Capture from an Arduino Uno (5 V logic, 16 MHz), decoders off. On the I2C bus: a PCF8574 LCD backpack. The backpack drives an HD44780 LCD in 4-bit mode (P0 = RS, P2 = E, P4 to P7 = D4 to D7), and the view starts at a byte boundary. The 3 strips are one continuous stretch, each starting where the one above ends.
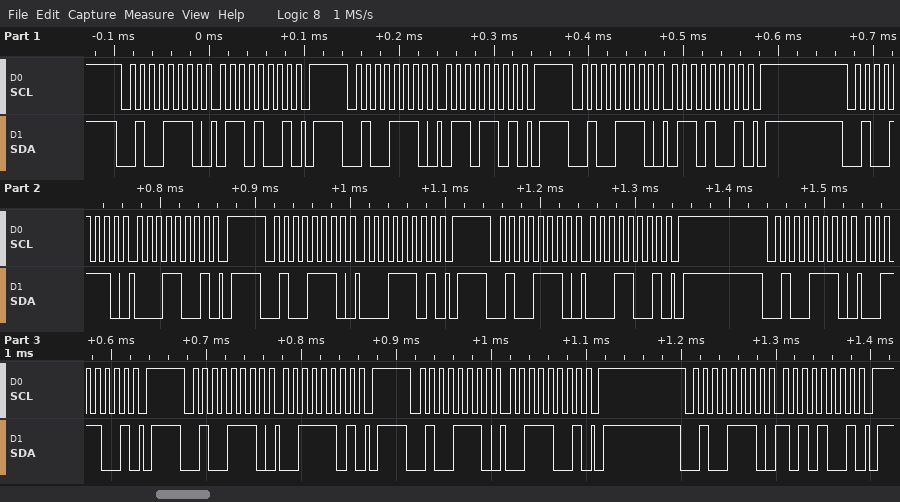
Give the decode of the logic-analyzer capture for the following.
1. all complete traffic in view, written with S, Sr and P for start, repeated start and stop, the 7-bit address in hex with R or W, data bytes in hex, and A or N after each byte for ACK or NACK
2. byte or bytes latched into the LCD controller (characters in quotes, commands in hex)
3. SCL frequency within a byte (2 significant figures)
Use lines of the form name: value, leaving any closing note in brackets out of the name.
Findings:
all complete traffic in view, written with S, Sr and P for start, repeated start and stop, the 7-bit address in hex with R or W, data bytes in hex, and A or N after each byte for ACK or NACK: S 27W A 69 A P S 27W A 6D A P S 27W A 69 A P S 27W A 19 A P S 27W A 1D A P S 27W A 19 A P S 27W A 39 A P S 27W A 3D A P S 27W A 39 A P S 27W A A9 A P
byte or bytes latched into the LCD controller: 'a'
SCL frequency within a byte: 100 kHz
